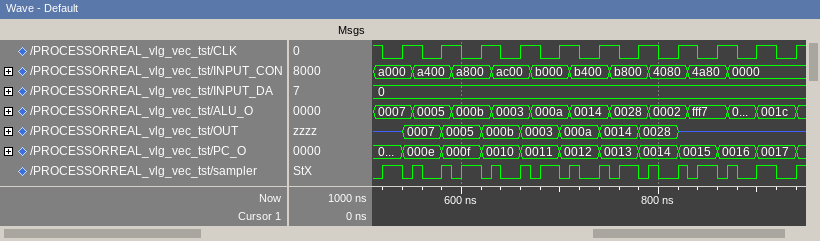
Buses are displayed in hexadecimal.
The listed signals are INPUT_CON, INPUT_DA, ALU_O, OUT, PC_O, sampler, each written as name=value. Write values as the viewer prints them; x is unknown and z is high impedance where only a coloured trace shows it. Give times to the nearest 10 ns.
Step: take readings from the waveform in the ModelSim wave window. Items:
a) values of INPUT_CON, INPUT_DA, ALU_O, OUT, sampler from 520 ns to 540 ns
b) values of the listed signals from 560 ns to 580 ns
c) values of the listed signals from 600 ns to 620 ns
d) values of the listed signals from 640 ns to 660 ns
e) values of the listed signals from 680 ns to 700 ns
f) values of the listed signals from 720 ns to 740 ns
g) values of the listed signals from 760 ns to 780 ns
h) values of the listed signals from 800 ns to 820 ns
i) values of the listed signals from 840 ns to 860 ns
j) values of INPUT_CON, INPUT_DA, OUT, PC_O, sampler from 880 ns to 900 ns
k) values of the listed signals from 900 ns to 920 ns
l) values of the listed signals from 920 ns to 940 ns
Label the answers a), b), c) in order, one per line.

a) INPUT_CON=a000, INPUT_DA=0, ALU_O=0007, OUT=z, sampler=1
b) INPUT_CON=a400, INPUT_DA=0, ALU_O=0005, OUT=0007, PC_O=000e, sampler=0
c) INPUT_CON=a800, INPUT_DA=0, ALU_O=000b, OUT=0005, PC_O=000f, sampler=1
d) INPUT_CON=ac00, INPUT_DA=0, ALU_O=0003, OUT=000b, PC_O=0010, sampler=0
e) INPUT_CON=b000, INPUT_DA=0, ALU_O=000a, OUT=0003, PC_O=0011, sampler=1
f) INPUT_CON=b400, INPUT_DA=0, ALU_O=0014, OUT=000a, PC_O=0012, sampler=0
g) INPUT_CON=b800, INPUT_DA=0, ALU_O=0028, OUT=0014, PC_O=0013, sampler=1
h) INPUT_CON=4080, INPUT_DA=0, ALU_O=0002, OUT=0028, PC_O=0014, sampler=0
i) INPUT_CON=4a80, INPUT_DA=0, ALU_O=fff7, OUT=z, PC_O=0015, sampler=1
j) INPUT_CON=0000, INPUT_DA=0, OUT=z, PC_O=0016, sampler=0
k) INPUT_CON=0000, INPUT_DA=0, ALU_O=001c, OUT=z, PC_O=0017, sampler=1
l) INPUT_CON=0000, INPUT_DA=0, ALU_O=001c, OUT=z, PC_O=0017, sampler=0
